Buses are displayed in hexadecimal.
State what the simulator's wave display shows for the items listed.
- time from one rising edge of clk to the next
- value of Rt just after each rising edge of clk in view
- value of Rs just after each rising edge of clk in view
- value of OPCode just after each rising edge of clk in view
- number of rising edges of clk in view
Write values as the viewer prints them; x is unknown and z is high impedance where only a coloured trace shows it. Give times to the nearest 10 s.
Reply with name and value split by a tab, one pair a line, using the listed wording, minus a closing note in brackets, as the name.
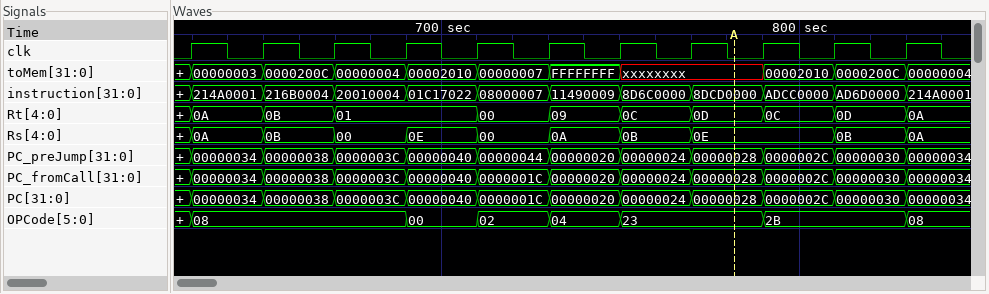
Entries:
time from one rising edge of clk to the next	20 s
value of Rt just after each rising edge of clk in view	0A, 0B, 01, 01, 00, 09, 0C, 0D, 0C, 0D, 0A
value of Rs just after each rising edge of clk in view	0A, 0B, 00, 0E, 00, 0A, 0B, 0E, 0E, 0B, 0A
value of OPCode just after each rising edge of clk in view	08, 08, 08, 00, 02, 04, 23, 23, 2B, 2B, 08
number of rising edges of clk in view	11
